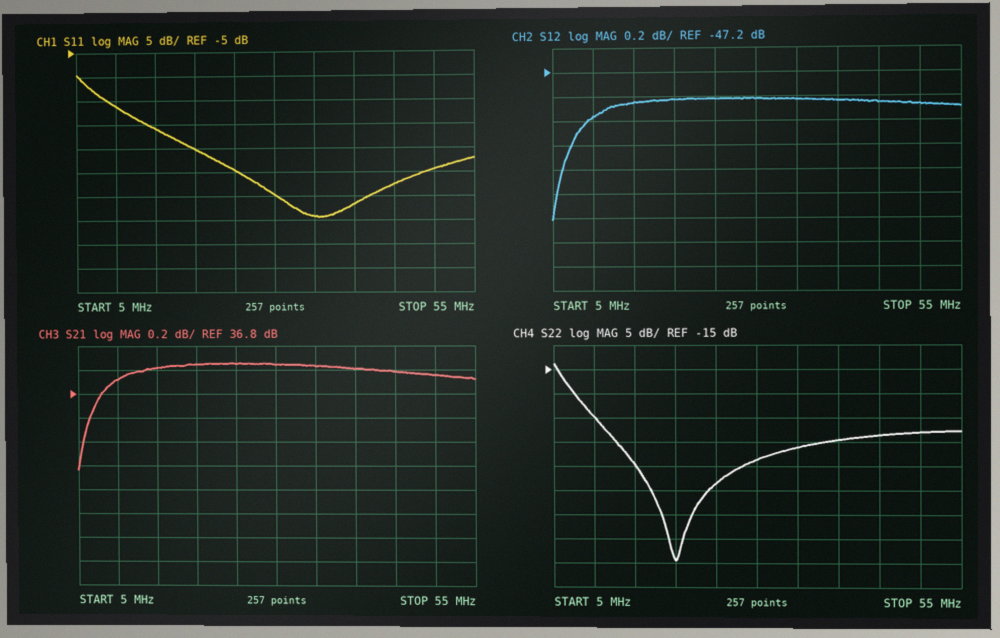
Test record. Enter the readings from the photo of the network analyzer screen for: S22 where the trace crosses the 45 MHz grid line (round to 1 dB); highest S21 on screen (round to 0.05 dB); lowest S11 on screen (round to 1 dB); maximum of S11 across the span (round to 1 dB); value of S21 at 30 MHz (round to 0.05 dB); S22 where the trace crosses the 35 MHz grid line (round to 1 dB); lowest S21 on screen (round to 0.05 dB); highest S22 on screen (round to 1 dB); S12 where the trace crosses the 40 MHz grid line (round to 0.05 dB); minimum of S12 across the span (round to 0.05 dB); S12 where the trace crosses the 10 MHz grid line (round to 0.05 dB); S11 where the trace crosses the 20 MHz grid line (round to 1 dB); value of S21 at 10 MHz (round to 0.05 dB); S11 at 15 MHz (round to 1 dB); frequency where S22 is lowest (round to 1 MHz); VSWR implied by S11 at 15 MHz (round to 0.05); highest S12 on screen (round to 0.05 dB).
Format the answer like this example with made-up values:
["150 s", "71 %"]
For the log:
["-29 dB", "37.05 dB", "-39 dB", "-10 dB", "37.05 dB", "-31 dB", "36.15 dB", "-14 dB", "-47.45 dB", "-48.40 dB", "-47.55 dB", "-25 dB", "36.90 dB", "-21 dB", "20 MHz", "1.20", "-47.40 dB"]
